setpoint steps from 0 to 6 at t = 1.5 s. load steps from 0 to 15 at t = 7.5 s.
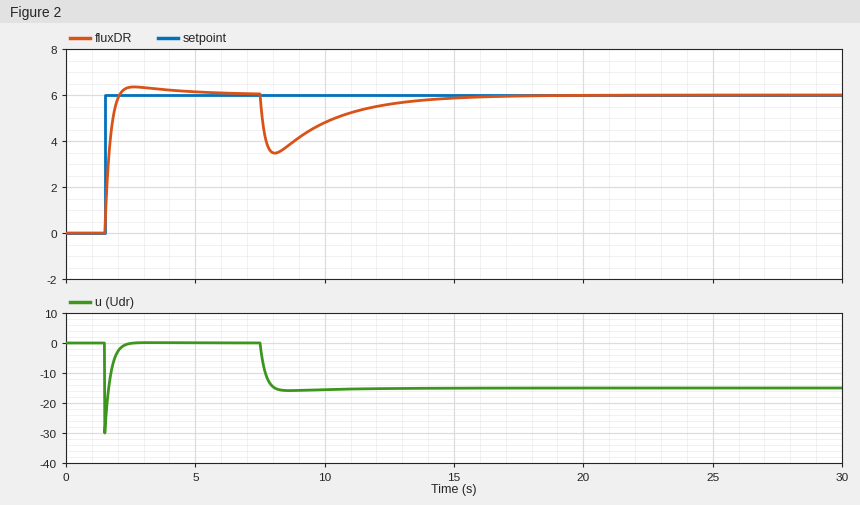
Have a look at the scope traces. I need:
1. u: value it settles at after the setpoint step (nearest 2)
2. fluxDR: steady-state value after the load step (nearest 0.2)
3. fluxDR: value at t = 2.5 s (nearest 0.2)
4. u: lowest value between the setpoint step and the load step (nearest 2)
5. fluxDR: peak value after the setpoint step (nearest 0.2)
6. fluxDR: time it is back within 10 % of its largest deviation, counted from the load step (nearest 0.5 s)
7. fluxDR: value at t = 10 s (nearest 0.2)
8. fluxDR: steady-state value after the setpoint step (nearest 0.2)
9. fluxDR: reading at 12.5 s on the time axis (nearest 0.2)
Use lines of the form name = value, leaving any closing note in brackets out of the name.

u: value it settles at after the setpoint step = 0
fluxDR: steady-state value after the load step = 6.0
fluxDR: value at t = 2.5 s = 6.4
u: lowest value between the setpoint step and the load step = -30
fluxDR: peak value after the setpoint step = 6.4
fluxDR: time it is back within 10 % of its largest deviation, counted from the load step = 6.0 s
fluxDR: value at t = 10 s = 4.8
fluxDR: steady-state value after the setpoint step = 6.0
fluxDR: reading at 12.5 s on the time axis = 5.6
